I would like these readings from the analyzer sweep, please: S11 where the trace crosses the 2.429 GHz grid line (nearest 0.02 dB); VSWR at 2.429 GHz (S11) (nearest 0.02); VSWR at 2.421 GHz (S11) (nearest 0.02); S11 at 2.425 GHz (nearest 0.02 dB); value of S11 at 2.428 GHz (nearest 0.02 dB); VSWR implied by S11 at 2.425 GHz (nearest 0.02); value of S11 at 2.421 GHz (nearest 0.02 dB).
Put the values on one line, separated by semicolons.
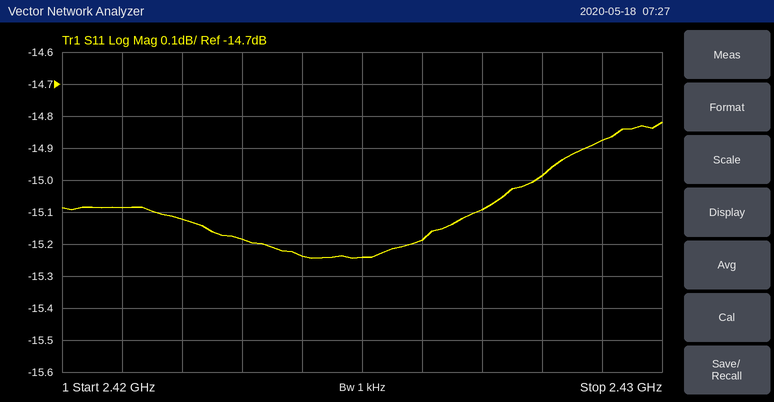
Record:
-14.88 dB; 1.44; 1.42; -15.24 dB; -14.98 dB; 1.42; -15.08 dB
